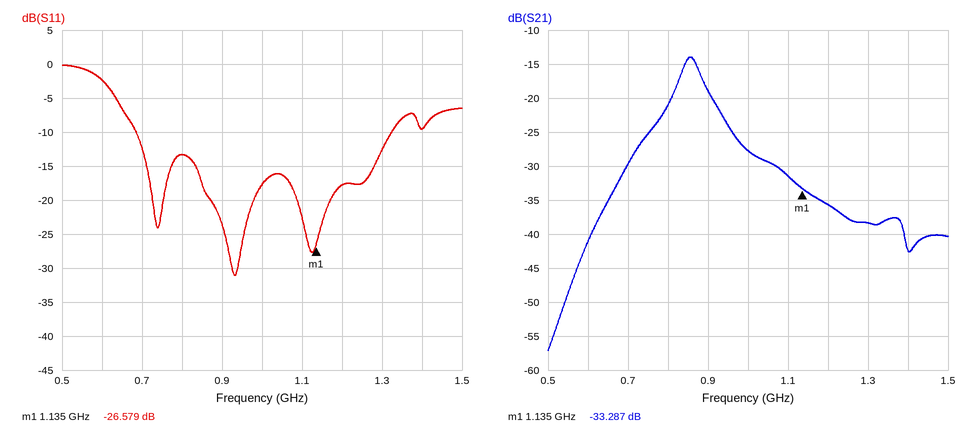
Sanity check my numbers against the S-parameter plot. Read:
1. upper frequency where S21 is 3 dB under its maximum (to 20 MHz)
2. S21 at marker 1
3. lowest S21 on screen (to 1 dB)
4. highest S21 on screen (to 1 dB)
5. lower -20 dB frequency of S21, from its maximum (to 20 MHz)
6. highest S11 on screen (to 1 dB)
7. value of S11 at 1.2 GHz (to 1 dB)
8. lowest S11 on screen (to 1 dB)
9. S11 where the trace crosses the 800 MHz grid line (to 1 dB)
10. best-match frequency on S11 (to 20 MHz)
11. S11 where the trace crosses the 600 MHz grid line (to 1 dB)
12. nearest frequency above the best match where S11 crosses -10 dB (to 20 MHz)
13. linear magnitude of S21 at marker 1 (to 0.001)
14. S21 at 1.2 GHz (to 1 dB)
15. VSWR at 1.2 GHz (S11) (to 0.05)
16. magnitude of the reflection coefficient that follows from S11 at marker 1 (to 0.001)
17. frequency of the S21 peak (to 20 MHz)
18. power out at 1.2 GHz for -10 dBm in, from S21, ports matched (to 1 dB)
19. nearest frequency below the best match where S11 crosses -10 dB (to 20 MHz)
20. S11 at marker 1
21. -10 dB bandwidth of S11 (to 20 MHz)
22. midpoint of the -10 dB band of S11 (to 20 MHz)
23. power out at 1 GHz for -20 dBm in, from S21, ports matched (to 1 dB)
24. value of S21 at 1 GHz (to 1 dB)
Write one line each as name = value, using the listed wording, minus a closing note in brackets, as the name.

upper frequency where S21 is 3 dB under its maximum = 880 MHz
S21 at marker 1 = -33.287 dB
lowest S21 on screen = -57 dB
highest S21 on screen = -14 dB
lower -20 dB frequency of S21, from its maximum = 660 MHz
highest S11 on screen = 0 dB
value of S11 at 1.2 GHz = -18 dB
lowest S11 on screen = -31 dB
S11 where the trace crosses the 800 MHz grid line = -13 dB
best-match frequency on S11 = 940 MHz
S11 where the trace crosses the 600 MHz grid line = -2 dB
nearest frequency above the best match where S11 crosses -10 dB = 1.32 GHz
linear magnitude of S21 at marker 1 = 0.022
S21 at 1.2 GHz = -36 dB
VSWR at 1.2 GHz (S11) = 1.30
magnitude of the reflection coefficient that follows from S11 at marker 1 = 0.047
frequency of the S21 peak = 860 MHz
power out at 1.2 GHz for -10 dBm in, from S21, ports matched = -46 dBm
nearest frequency below the best match where S11 crosses -10 dB = 680 MHz
S11 at marker 1 = -26.579 dB
-10 dB bandwidth of S11 = 640 MHz
midpoint of the -10 dB band of S11 = 1.00 GHz
power out at 1 GHz for -20 dBm in, from S21, ports matched = -48 dBm
value of S21 at 1 GHz = -28 dB
